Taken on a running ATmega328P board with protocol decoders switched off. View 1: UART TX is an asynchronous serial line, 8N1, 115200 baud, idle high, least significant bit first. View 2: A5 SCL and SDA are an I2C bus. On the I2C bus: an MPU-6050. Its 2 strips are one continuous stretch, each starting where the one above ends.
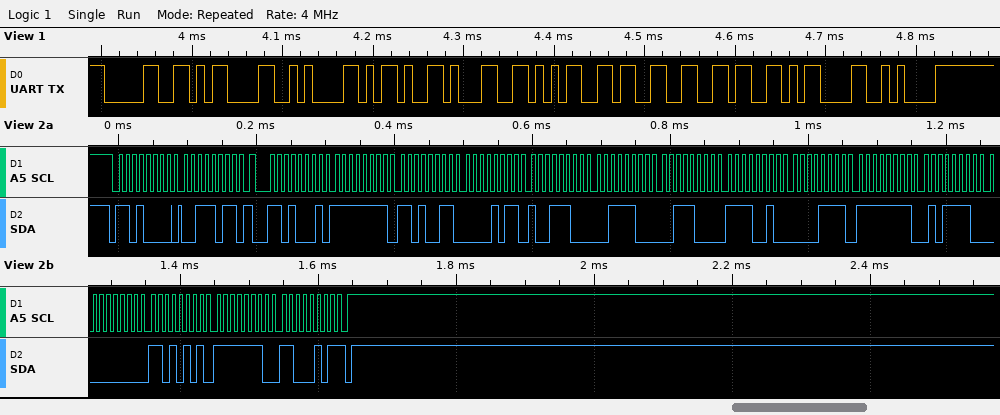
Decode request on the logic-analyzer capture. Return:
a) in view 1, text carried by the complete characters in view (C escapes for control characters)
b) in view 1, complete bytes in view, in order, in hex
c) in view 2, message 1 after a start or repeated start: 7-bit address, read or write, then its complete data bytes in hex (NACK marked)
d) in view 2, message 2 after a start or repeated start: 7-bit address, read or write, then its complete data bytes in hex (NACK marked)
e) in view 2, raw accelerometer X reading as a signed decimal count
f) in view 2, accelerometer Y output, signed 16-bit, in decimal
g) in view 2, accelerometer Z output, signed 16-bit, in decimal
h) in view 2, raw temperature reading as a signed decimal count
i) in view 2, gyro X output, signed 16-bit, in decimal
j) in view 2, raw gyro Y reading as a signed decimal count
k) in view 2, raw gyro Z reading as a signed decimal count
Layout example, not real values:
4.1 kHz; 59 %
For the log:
"0\r\n-1536\r\n"; 30 0D 0A 2D 31 35 33 36 0D 0A; 0x68 write: 3B; 0x68 read: FF D3 0B 9C 3C 38 F2 0F FF 5E 00 D5 FE C5 NACK; -45; 2972; 15416; -3569; -162; 213; -315
